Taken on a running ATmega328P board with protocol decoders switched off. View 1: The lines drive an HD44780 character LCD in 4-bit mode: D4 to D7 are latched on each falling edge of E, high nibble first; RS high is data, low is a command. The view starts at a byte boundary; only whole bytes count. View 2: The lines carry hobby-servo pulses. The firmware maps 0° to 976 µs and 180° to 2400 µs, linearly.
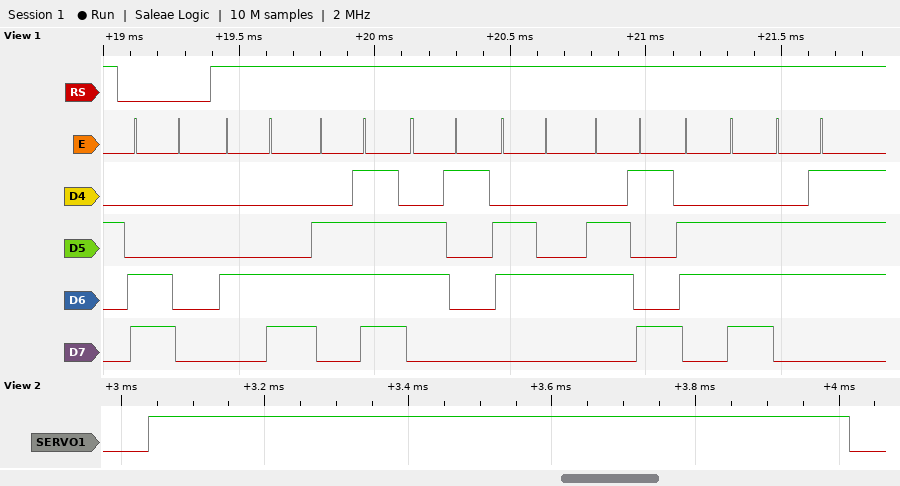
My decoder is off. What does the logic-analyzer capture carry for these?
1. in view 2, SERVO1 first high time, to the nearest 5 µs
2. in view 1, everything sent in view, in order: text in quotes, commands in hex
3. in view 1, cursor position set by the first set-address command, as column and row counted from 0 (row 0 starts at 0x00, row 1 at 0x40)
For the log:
975 µs
0xC0 "Loading"
column 0, row 1
